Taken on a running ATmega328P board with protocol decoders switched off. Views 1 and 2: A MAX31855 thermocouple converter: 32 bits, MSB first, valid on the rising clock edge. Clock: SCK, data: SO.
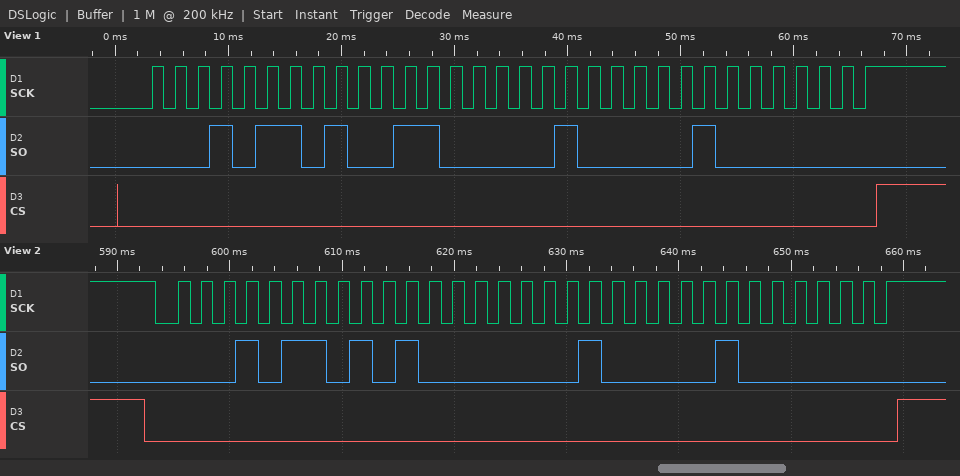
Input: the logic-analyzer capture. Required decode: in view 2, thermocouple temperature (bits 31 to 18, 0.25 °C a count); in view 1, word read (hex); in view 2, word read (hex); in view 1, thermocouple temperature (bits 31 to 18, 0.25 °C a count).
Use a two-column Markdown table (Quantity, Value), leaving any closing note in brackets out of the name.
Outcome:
| Quantity | Value |
|---|---|
| in view 2, thermocouple temperature | 362.00 °C |
| in view 1, word read | 0x16982080 |
| in view 2, word read | 0x16A02080 |
| in view 1, thermocouple temperature | 361.50 °C |
